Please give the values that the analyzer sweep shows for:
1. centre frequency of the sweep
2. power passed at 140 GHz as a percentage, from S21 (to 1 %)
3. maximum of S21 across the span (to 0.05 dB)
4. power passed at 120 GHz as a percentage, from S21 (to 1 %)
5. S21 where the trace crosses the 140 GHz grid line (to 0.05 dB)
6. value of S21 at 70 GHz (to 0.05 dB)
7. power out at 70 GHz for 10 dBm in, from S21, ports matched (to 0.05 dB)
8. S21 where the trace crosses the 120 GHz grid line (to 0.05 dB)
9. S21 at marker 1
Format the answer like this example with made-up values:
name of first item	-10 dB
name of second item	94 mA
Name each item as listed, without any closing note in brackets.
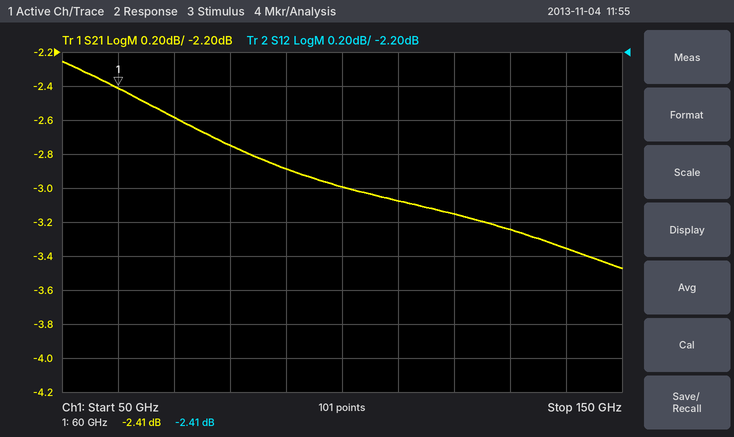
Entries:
centre frequency of the sweep	100 GHz
power passed at 140 GHz as a percentage, from S21	46 %
maximum of S21 across the span	-2.25 dB
power passed at 120 GHz as a percentage, from S21	48 %
S21 where the trace crosses the 140 GHz grid line	-3.35 dB
value of S21 at 70 GHz	-2.60 dB
power out at 70 GHz for 10 dBm in, from S21, ports matched	7.40 dBm
S21 where the trace crosses the 120 GHz grid line	-3.15 dB
S21 at marker 1	-2.41 dB
